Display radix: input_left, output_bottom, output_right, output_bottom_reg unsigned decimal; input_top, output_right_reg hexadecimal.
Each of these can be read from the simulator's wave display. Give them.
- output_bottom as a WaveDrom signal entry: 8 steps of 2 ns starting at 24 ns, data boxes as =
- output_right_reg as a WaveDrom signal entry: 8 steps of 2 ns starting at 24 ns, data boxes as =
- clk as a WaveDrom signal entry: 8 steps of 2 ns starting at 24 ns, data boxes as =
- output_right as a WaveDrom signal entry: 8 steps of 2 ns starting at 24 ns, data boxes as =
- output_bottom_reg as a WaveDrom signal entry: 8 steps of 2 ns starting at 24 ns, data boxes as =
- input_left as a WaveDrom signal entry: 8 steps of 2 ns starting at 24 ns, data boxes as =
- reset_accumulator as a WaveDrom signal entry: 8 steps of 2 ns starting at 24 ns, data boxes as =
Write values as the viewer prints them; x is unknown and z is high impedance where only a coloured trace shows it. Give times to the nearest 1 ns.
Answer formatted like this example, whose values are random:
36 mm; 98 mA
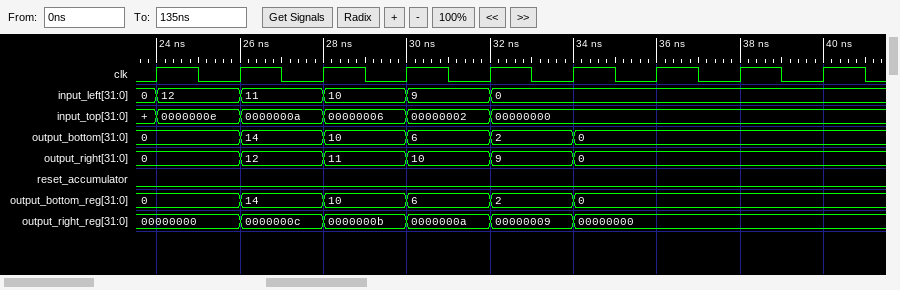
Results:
{name: 'output_bottom', wave: '======..', data: '0 14 10 6 2 0'}; {name: 'output_right_reg', wave: '======..', data: '00000000 0000000c 0000000b 0000000a 00000009 00000000'}; {name: 'clk', wave: 'p.......'}; {name: 'output_right', wave: '======..', data: '0 12 11 10 9 0'}; {name: 'output_bottom_reg', wave: '======..', data: '0 14 10 6 2 0'}; {name: 'input_left', wave: '=====...', data: '12 11 10 9 0'}; {name: 'reset_accumulator', wave: '0.......'}
